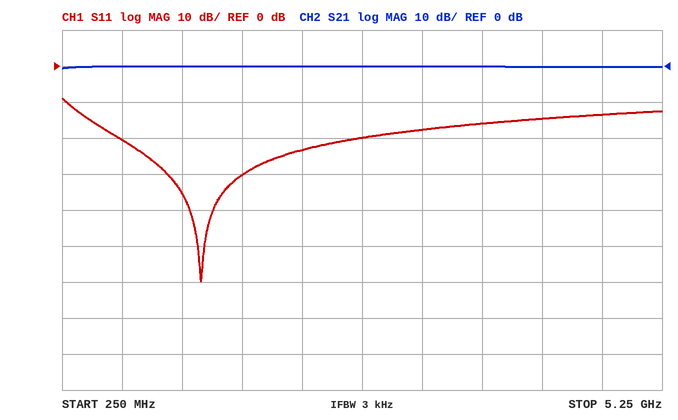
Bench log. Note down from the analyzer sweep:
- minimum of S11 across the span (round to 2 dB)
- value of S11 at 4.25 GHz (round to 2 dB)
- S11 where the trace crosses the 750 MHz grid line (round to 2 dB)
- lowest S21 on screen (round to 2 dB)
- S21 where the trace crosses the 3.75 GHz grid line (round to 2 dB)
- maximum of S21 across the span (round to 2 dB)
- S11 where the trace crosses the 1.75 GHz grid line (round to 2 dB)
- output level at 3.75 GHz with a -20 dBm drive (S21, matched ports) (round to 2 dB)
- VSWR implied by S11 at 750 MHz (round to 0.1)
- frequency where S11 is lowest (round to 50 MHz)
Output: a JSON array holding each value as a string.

["-60 dB", "-14 dB", "-20 dB", "0 dB", "0 dB", "0 dB", "-30 dB", "-20 dBm", "1.2", "1.40 GHz"]
